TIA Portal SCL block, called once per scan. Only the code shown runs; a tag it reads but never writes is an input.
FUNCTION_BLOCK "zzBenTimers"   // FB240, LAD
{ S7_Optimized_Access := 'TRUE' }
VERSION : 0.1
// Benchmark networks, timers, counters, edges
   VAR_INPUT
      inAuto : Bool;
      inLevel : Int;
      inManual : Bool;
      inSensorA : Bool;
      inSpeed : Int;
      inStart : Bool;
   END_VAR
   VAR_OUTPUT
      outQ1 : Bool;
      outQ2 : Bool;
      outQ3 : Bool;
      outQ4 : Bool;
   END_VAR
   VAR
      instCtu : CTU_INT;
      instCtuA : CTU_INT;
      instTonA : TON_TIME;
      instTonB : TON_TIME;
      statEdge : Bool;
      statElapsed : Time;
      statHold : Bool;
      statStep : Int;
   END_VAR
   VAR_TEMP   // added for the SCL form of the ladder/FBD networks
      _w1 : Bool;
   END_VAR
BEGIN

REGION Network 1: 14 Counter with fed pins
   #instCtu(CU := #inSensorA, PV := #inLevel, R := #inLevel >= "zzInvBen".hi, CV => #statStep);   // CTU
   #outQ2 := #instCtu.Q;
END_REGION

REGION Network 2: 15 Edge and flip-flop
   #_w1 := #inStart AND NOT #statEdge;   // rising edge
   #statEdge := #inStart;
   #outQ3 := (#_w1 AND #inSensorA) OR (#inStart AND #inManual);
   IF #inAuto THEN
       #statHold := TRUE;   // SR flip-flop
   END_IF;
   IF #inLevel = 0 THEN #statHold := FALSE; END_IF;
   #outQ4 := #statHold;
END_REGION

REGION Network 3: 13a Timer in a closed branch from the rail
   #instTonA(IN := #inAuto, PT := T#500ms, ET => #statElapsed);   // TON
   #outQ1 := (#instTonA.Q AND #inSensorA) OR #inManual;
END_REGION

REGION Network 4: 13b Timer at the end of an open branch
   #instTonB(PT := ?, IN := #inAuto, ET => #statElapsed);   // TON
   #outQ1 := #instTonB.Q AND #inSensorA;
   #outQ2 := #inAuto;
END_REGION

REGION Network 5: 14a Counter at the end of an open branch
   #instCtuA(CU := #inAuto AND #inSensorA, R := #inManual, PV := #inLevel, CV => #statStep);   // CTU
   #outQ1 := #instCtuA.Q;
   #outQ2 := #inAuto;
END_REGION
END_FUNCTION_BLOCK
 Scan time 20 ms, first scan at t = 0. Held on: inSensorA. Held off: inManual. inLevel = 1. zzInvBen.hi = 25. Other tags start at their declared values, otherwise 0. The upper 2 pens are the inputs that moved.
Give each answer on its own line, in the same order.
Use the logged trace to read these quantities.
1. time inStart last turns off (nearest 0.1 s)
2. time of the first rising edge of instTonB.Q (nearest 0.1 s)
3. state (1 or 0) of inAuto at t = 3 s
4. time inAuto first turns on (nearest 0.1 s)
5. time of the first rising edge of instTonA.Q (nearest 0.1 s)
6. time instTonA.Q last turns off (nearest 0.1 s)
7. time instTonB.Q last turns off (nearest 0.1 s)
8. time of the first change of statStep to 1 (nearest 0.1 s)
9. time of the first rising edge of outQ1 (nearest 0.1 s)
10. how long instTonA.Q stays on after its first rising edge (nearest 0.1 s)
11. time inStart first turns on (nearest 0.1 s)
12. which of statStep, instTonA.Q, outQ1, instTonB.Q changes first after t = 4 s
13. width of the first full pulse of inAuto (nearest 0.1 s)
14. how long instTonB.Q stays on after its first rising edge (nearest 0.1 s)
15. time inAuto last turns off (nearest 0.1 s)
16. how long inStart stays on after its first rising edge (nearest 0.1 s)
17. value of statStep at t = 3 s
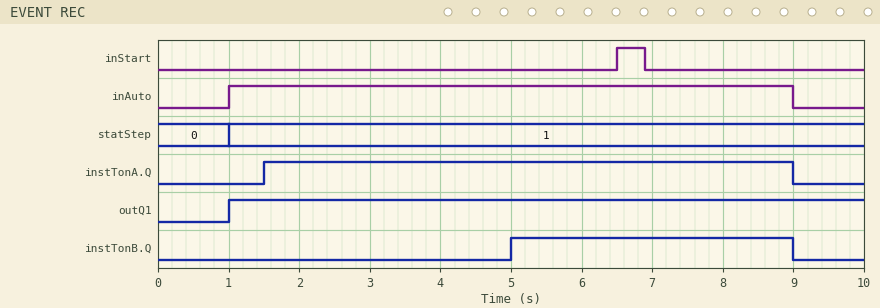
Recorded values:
6.9 s
5.0 s
1
1.0 s
1.5 s
9.0 s
9.0 s
1.0 s
1.0 s
7.5 s
6.5 s
instTonB.Q
8.0 s
4.0 s
9.0 s
0.4 s
1
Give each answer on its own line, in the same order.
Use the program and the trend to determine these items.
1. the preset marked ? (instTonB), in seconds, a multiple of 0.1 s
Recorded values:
4.0 s
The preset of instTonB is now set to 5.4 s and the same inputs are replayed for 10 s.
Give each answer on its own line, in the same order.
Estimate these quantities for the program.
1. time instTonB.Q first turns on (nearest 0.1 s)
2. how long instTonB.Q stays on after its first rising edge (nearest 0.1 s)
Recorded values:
6.4 s
2.6 s
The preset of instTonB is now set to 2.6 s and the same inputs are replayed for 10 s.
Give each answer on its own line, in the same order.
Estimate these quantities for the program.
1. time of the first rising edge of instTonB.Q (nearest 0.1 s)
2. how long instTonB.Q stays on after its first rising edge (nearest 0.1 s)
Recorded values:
3.6 s
5.4 s
